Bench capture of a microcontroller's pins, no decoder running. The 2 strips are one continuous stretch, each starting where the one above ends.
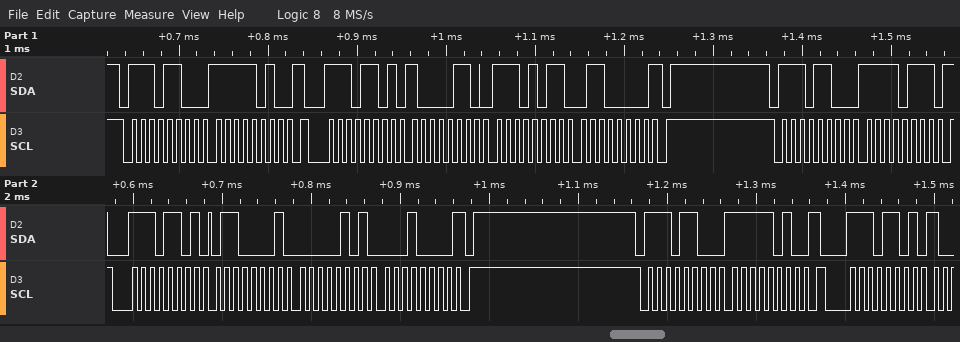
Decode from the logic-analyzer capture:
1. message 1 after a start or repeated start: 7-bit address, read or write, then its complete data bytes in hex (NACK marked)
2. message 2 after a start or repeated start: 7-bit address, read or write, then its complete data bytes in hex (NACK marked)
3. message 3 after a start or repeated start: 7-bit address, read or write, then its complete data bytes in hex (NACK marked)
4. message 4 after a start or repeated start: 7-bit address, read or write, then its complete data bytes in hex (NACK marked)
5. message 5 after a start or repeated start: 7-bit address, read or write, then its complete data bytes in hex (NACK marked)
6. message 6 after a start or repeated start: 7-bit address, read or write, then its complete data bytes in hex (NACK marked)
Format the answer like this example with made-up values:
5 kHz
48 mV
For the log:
0x76 write: FA
0x76 read: 86 EB 60 NACK
0x76 write: F7
0x76 read: 61 05 10 NACK
0x76 write: FA
0x76 read
